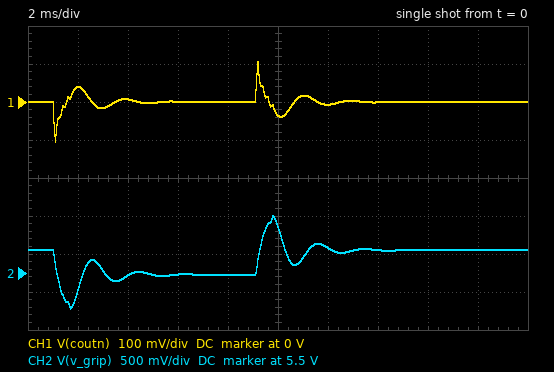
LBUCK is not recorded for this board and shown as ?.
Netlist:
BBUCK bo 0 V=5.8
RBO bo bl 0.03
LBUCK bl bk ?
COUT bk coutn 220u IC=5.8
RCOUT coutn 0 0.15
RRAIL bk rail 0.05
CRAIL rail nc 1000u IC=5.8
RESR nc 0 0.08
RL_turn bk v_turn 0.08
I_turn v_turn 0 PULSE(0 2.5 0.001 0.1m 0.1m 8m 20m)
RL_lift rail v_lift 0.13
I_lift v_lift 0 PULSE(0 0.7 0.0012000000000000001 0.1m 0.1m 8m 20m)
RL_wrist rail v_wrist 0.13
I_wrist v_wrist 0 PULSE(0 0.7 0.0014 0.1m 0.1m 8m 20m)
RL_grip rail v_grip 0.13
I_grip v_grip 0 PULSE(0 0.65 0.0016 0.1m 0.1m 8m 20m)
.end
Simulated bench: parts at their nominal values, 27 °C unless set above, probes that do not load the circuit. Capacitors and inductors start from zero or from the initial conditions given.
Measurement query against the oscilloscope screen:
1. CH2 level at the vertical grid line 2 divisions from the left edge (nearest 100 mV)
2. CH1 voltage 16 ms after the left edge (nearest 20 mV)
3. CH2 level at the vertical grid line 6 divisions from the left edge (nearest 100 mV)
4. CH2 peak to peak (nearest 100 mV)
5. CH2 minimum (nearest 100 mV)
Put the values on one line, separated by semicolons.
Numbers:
5.5 V; 0 V; 5.8 V; 1.2 V; 5.0 V
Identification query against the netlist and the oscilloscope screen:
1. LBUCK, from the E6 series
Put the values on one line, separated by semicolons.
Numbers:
68 µH
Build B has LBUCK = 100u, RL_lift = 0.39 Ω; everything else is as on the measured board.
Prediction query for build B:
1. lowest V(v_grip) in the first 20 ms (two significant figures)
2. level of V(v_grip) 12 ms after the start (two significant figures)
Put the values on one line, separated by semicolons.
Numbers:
4.8 V; 6.0 V
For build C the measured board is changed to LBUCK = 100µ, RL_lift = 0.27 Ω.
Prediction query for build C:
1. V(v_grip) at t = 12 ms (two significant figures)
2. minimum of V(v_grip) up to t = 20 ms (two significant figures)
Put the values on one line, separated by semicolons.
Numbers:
6.0 V; 4.8 V
